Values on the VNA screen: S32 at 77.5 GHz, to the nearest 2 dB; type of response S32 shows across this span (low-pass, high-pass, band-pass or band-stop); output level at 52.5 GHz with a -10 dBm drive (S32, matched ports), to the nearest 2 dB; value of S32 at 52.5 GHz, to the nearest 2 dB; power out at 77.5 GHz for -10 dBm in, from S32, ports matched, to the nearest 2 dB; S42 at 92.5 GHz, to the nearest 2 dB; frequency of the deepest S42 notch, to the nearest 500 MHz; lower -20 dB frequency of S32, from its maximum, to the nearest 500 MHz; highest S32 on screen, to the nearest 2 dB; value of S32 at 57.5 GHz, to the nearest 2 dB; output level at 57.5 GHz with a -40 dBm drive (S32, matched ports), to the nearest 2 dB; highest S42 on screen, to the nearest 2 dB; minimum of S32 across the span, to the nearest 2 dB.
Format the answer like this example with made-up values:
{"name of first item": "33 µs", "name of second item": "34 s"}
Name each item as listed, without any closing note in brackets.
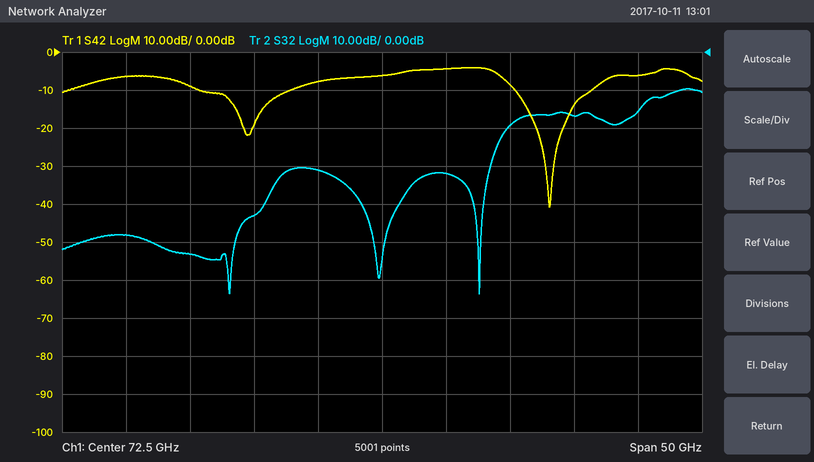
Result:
{"S32 at 77.5 GHz, to the nearest 2 dB": "-32 dB", "type of response S32 shows across this span": "high-pass", "output level at 52.5 GHz with a -10 dBm drive (S32, matched ports), to the nearest 2 dB": "-58 dBm", "value of S32 at 52.5 GHz, to the nearest 2 dB": "-48 dB", "power out at 77.5 GHz for -10 dBm in, from S32, ports matched, to the nearest 2 dB": "-42 dBm", "S42 at 92.5 GHz, to the nearest 2 dB": "-6 dB", "frequency of the deepest S42 notch, to the nearest 500 MHz": "85.5 GHz", "lower -20 dB frequency of S32, from its maximum, to the nearest 500 MHz": "81.0 GHz", "highest S32 on screen, to the nearest 2 dB": "-10 dB", "value of S32 at 57.5 GHz, to the nearest 2 dB": "-54 dB", "output level at 57.5 GHz with a -40 dBm drive (S32, matched ports), to the nearest 2 dB": "-94 dBm", "highest S42 on screen, to the nearest 2 dB": "-4 dB", "minimum of S32 across the span, to the nearest 2 dB": "-64 dB"}
